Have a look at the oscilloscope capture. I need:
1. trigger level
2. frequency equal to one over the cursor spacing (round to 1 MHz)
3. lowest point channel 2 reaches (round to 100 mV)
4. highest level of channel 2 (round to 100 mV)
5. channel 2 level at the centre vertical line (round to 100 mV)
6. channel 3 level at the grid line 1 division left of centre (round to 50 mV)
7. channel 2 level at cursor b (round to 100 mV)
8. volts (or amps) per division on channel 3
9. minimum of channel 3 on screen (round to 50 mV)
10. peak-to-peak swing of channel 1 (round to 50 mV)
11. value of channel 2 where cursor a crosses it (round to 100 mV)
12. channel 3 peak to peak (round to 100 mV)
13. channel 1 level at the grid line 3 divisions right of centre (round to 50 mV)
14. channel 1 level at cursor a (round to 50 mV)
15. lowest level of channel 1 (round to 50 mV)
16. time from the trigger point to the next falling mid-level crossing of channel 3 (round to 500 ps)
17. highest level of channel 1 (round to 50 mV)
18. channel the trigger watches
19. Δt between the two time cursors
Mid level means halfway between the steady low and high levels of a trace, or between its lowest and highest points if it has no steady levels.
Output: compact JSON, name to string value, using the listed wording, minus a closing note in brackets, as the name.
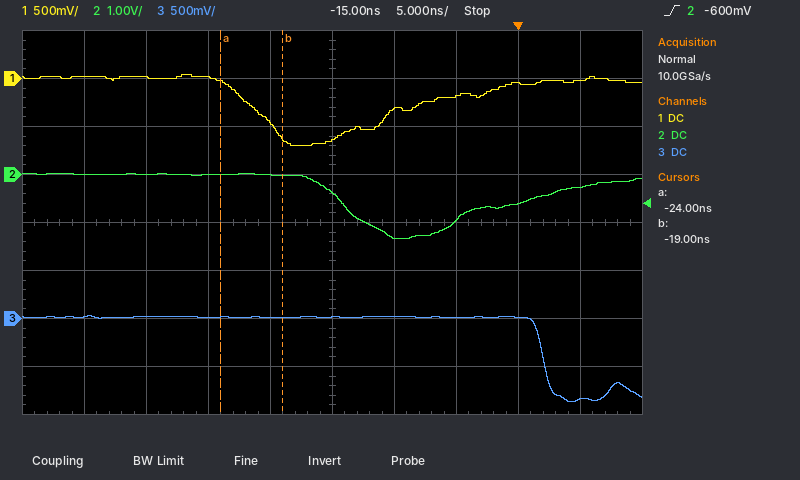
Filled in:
{"trigger level": "-600 mV", "frequency equal to one over the cursor spacing": "200 MHz", "lowest point channel 2 reaches": "-1.3 V", "highest level of channel 2": "0.0 V", "channel 2 level at the centre vertical line": "-400 mV", "channel 3 level at the grid line 1 division left of centre": "0 mV", "channel 2 level at cursor b": "0.0 V", "volts (or amps) per division on channel 3": "500 mV", "minimum of channel 3 on screen": "-850 mV", "peak-to-peak swing of channel 1": "750 mV", "value of channel 2 where cursor a crosses it": "0.0 V", "channel 3 peak to peak": "900 mV", "channel 1 level at the grid line 3 divisions right of centre": "-50 mV", "channel 1 level at cursor a": "-50 mV", "lowest level of channel 1": "-700 mV", "time from the trigger point to the next falling mid-level crossing of channel 3": "2.0 ns", "highest level of channel 1": "50 mV", "channel the trigger watches": "channel 2", "Δt between the two time cursors": "5.0 ns"}
